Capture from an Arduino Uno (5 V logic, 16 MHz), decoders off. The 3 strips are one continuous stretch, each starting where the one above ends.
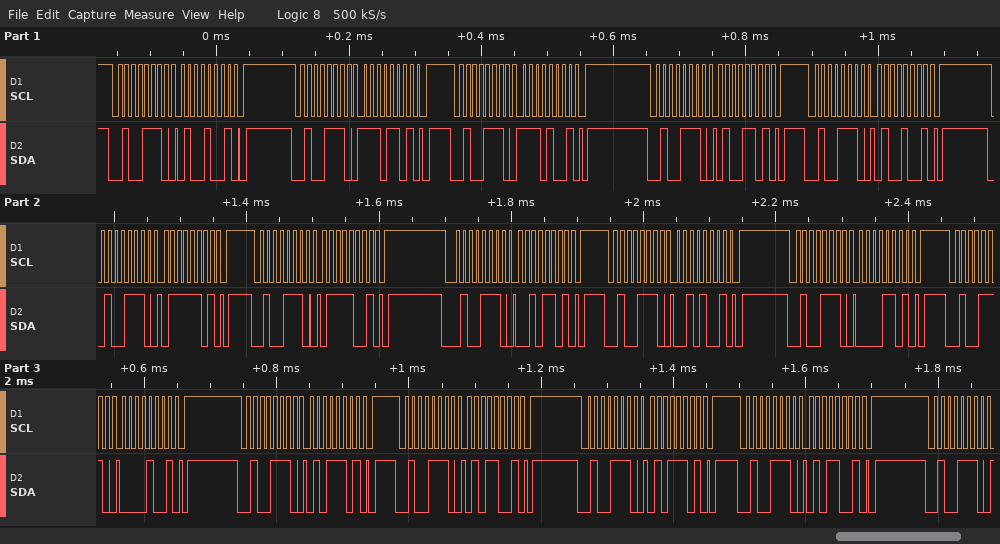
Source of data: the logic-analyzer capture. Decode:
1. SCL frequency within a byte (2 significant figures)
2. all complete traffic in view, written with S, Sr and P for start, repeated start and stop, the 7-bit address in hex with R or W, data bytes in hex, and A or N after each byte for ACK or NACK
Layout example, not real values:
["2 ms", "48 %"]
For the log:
["100 kHz", "S 27W A 49 A P S 27W A ED A P S 27W A E9 A P S 27W A 4D A P S 27W A 49 A P S 27W A 7D A P S 27W A 79 A P S 27W A 2D A P S 27W A 29 A P S 27W A 0D A P S 27W A 09 A P S 27W A 5D A P S 27W A 59 A P S 27W A 5D A P S 27W A 59 A P S 27W A"]
